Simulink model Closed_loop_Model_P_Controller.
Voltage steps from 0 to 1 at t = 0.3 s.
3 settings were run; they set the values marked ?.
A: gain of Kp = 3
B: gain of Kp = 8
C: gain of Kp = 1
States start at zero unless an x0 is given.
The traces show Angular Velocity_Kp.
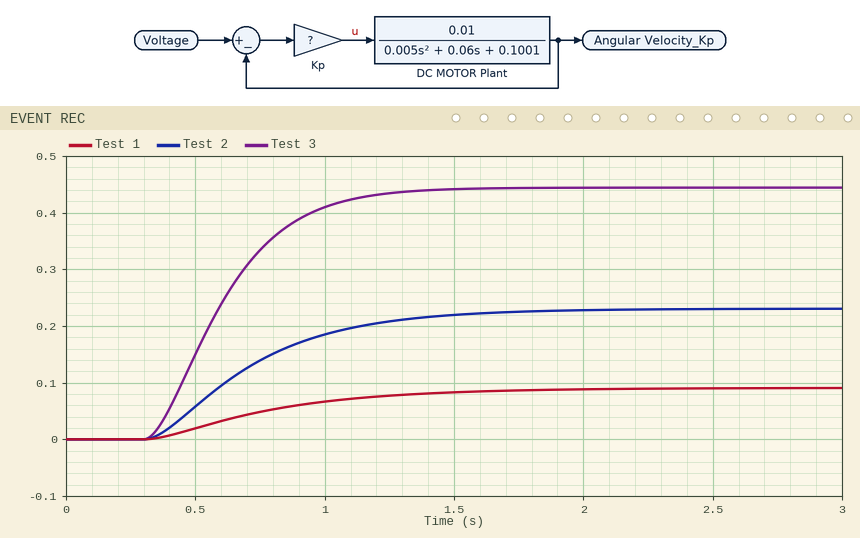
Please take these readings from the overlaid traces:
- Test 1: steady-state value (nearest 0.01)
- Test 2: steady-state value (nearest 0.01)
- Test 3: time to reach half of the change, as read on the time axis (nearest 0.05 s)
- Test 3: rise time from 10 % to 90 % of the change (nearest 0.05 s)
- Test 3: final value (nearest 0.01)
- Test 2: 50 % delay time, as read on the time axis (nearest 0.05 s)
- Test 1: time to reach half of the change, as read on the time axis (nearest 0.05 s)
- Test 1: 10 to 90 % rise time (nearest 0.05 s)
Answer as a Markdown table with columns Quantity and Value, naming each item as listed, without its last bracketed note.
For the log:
| Quantity | Value |
|---|---|
| Test 1: steady-state value | 0.09 |
| Test 2: steady-state value | 0.23 |
| Test 3: time to reach half of the change, as read on the time axis | 0.60 s |
| Test 3: rise time from 10 % to 90 % of the change | 0.55 s |
| Test 3: final value | 0.44 |
| Test 2: 50 % delay time, as read on the time axis | 0.65 s |
| Test 1: time to reach half of the change, as read on the time axis | 0.70 s |
| Test 1: 10 to 90 % rise time | 1.00 s |
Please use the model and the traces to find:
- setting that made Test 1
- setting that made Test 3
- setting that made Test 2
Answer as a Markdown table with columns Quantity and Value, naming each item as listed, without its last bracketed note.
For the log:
| Quantity | Value |
|---|---|
| setting that made Test 1 | C |
| setting that made Test 3 | B |
| setting that made Test 2 | A |
